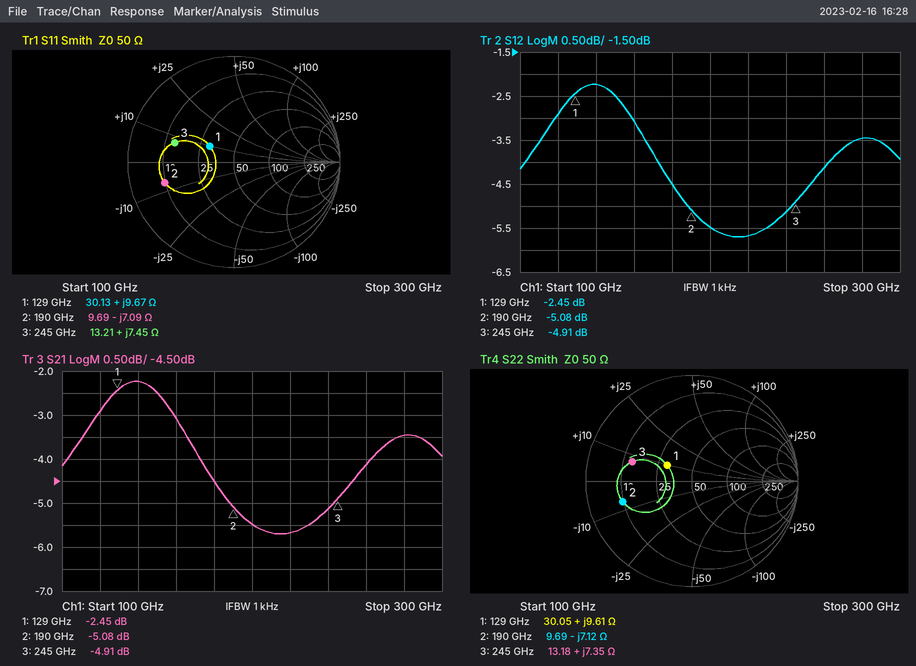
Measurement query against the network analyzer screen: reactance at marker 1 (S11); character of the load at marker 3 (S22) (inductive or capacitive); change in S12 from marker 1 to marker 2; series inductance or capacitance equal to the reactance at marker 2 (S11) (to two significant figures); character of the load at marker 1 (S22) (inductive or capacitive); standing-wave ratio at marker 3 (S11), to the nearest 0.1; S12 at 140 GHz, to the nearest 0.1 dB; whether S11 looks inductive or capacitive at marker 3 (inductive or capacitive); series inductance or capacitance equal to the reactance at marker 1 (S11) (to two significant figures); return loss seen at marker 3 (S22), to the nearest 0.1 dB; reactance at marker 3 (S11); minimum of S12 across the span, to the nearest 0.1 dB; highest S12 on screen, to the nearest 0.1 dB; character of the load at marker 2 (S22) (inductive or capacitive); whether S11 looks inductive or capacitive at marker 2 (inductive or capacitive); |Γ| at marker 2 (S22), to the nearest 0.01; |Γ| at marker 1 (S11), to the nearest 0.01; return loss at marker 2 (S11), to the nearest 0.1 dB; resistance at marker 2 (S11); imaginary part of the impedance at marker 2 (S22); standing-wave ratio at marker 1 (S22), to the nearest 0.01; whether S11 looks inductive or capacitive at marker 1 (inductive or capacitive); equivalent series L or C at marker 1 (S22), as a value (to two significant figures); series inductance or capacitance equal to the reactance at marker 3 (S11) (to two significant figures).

+9.67 Ω
inductive
-2.63 dB
120 fF
inductive
3.9
-2.2 dB
inductive
12 pH
4.6 dB
+7.45 Ω
-5.7 dB
-2.2 dB
capacitive
capacitive
0.68
0.27
3.3 dB
9.69 Ω
-7.12 Ω
1.76
inductive
12 pH
4.8 pH
